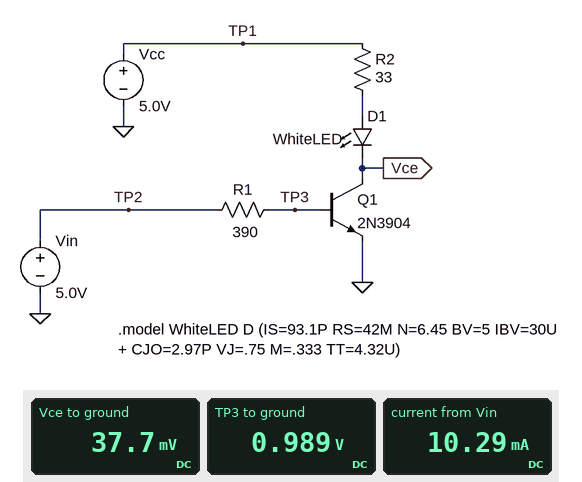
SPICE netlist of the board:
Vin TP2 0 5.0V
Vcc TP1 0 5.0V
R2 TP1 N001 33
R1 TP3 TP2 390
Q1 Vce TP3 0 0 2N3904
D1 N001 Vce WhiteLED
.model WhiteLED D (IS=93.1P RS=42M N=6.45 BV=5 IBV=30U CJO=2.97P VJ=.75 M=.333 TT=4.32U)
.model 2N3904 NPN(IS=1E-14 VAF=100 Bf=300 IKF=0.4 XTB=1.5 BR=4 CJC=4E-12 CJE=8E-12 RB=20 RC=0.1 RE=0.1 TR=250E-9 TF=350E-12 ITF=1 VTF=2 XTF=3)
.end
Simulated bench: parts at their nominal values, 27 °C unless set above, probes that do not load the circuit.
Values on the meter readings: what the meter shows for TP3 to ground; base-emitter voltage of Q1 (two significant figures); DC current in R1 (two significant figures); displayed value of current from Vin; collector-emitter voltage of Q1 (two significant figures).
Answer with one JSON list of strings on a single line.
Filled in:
["0.989 V", "990 mV", "10 mA", "10.29 mA", "38 mV"]
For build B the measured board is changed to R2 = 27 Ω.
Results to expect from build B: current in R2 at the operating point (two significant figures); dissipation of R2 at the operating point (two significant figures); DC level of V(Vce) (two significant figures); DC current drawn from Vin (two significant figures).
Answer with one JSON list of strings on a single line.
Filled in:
["58 mA", "92 mW", "43 mV", "10 mA"]
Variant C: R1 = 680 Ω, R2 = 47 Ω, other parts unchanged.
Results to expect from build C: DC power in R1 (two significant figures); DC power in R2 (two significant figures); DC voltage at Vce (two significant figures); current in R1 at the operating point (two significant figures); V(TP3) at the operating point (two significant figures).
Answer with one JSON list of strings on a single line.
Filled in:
["25 mW", "59 mW", "37 mV", "6.0 mA", "890 mV"]
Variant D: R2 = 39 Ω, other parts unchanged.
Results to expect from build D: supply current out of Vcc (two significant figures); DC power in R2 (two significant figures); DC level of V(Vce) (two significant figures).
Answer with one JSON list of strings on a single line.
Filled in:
["42 mA", "69 mW", "34 mV"]
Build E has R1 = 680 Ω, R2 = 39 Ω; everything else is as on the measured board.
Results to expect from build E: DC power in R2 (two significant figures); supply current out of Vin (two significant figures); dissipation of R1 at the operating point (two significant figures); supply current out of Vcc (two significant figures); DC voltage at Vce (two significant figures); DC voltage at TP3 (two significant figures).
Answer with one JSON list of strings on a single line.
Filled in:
["68 mW", "6.0 mA", "25 mW", "42 mA", "41 mV", "890 mV"]
